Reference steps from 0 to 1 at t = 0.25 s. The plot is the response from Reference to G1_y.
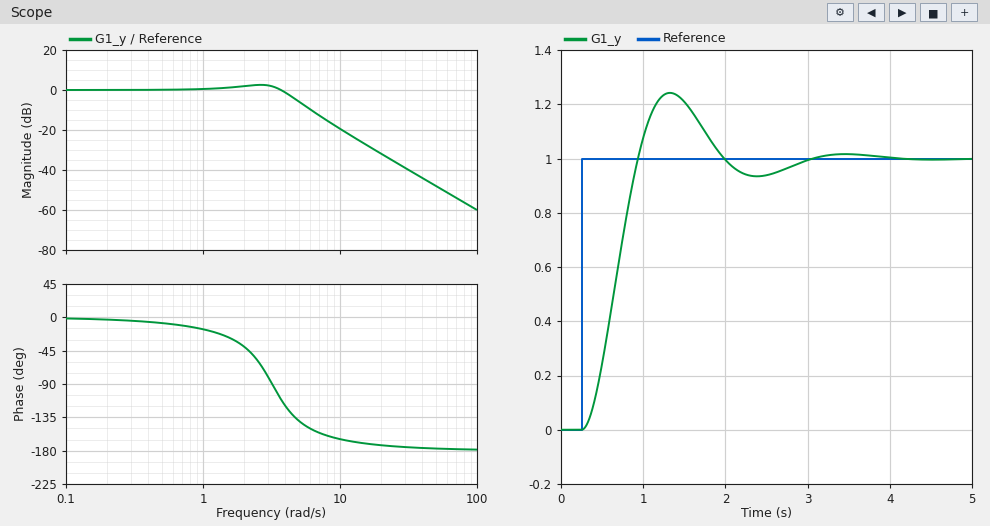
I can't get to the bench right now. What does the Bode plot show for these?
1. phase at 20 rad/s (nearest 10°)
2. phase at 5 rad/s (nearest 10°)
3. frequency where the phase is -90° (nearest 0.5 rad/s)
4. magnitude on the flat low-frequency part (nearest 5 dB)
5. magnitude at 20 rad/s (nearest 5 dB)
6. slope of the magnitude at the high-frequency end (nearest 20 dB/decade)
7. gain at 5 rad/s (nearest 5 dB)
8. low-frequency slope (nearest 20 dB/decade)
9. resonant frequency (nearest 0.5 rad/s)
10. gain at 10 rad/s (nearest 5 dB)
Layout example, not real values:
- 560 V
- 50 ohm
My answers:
- -170°
- -140°
- 3.0 rad/s
- 0 dB
- -30 dB
- -40 dB/decade
- -5 dB
- 0 dB/decade
- 2.5 rad/s
- -20 dB
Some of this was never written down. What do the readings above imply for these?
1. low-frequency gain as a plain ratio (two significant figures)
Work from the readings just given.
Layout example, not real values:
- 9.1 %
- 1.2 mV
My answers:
- 1.0
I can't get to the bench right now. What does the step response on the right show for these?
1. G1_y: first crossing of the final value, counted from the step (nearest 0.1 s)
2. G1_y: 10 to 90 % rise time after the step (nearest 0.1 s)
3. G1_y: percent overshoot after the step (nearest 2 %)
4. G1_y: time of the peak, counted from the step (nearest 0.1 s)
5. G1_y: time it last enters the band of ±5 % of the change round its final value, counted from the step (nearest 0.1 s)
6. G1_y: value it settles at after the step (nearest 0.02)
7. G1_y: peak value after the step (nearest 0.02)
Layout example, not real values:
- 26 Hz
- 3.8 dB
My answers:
- 0.7 s
- 0.5 s
- 24 %
- 1.1 s
- 2.4 s
- 1.00
- 1.24
